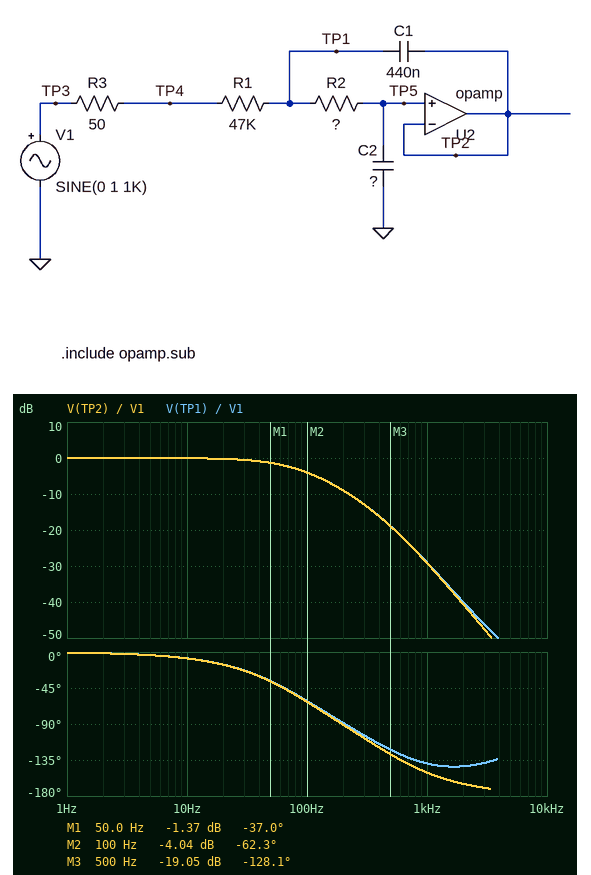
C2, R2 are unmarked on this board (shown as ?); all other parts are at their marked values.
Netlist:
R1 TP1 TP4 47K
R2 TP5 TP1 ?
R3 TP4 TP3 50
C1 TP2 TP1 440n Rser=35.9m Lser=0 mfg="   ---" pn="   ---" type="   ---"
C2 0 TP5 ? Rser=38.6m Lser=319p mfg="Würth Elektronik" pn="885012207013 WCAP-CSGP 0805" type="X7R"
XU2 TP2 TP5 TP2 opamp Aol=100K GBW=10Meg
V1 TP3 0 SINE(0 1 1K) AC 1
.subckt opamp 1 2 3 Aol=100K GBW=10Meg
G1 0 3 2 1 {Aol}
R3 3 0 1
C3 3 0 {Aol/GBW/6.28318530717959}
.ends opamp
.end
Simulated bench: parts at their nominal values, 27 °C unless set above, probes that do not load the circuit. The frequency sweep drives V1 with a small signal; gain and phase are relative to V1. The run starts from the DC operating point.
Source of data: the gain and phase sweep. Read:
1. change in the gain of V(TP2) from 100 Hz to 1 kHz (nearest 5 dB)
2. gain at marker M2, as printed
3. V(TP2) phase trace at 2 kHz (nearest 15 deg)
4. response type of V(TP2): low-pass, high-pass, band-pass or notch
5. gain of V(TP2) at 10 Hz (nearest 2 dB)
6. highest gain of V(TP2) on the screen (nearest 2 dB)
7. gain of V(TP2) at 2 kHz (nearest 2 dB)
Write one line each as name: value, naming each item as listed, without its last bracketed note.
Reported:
change in the gain of V(TP2) from 100 Hz to 1 kHz: -25 dB
gain at marker M2, as printed: -4.04 dB
V(TP2) phase trace at 2 kHz: -165 deg
response type of V(TP2): low-pass, high-pass, band-pass or notch: low-pass
gain of V(TP2) at 10 Hz: 0 dB
highest gain of V(TP2) on the screen: 0 dB
gain of V(TP2) at 2 kHz: -40 dB
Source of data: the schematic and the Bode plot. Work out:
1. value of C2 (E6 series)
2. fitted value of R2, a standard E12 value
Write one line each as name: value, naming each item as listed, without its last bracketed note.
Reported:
value of C2: 47 nF
fitted value of R2, a standard E12 value: 680 Ω
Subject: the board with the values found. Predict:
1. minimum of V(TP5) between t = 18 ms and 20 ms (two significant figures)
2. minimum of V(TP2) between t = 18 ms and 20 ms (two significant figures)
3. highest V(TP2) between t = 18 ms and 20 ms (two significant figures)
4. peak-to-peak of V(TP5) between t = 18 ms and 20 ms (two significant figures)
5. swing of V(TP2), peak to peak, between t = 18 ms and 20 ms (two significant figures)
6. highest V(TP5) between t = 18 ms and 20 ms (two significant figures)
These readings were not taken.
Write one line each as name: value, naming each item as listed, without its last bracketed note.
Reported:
minimum of V(TP5) between t = 18 ms and 20 ms: -35 mV
minimum of V(TP2) between t = 18 ms and 20 ms: -35 mV
highest V(TP2) between t = 18 ms and 20 ms: 35 mV
peak-to-peak of V(TP5) between t = 18 ms and 20 ms: 69 mV
swing of V(TP2), peak to peak, between t = 18 ms and 20 ms: 69 mV
highest V(TP5) between t = 18 ms and 20 ms: 35 mV
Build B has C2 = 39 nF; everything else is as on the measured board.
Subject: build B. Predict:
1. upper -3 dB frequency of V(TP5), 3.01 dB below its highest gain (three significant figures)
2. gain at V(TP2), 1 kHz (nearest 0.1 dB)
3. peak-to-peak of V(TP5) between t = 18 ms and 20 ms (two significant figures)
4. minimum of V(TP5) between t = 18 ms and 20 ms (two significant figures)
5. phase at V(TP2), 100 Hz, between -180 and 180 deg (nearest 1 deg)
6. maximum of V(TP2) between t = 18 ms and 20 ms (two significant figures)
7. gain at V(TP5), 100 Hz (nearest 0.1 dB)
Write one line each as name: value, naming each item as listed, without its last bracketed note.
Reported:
upper -3 dB frequency of V(TP5), 3.01 dB below its highest gain: 101 Hz
gain at V(TP2), 1 kHz: -27.5 dB
peak-to-peak of V(TP5) between t = 18 ms and 20 ms: 84 mV
minimum of V(TP5) between t = 18 ms and 20 ms: -42 mV
phase at V(TP2), 100 Hz, between -180 and 180 deg: -56 deg
maximum of V(TP2) between t = 18 ms and 20 ms: 42 mV
gain at V(TP5), 100 Hz: -3.0 dB
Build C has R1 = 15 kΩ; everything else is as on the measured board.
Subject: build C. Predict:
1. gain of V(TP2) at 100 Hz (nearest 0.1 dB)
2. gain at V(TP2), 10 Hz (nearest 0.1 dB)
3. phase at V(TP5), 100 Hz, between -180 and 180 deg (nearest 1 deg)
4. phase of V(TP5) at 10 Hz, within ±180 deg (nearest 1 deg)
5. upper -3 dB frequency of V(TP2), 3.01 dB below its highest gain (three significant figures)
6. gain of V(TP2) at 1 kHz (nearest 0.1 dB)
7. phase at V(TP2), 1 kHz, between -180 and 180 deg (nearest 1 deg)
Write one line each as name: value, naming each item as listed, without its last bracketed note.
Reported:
gain of V(TP2) at 100 Hz: -0.2 dB
gain at V(TP2), 10 Hz: 0 dB
phase at V(TP5), 100 Hz, between -180 and 180 deg: -27 deg
phase of V(TP5) at 10 Hz, within ±180 deg: -3 deg
upper -3 dB frequency of V(TP2), 3.01 dB below its highest gain: 300 Hz
gain of V(TP2) at 1 kHz: -18.8 dB
phase at V(TP2), 1 kHz, between -180 and 180 deg: -148 deg
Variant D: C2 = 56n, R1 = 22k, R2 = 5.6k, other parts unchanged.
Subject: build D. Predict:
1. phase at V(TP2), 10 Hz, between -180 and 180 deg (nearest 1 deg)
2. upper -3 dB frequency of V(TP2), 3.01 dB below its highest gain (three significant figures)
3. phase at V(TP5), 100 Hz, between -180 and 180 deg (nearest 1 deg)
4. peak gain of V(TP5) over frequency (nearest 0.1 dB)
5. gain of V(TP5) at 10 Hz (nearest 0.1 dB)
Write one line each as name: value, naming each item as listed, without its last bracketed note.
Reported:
phase at V(TP2), 10 Hz, between -180 and 180 deg: -6 deg
upper -3 dB frequency of V(TP2), 3.01 dB below its highest gain: 108 Hz
phase at V(TP5), 100 Hz, between -180 and 180 deg: -102 deg
peak gain of V(TP5) over frequency: 2.0 dB
gain of V(TP5) at 10 Hz: 0.1 dB
